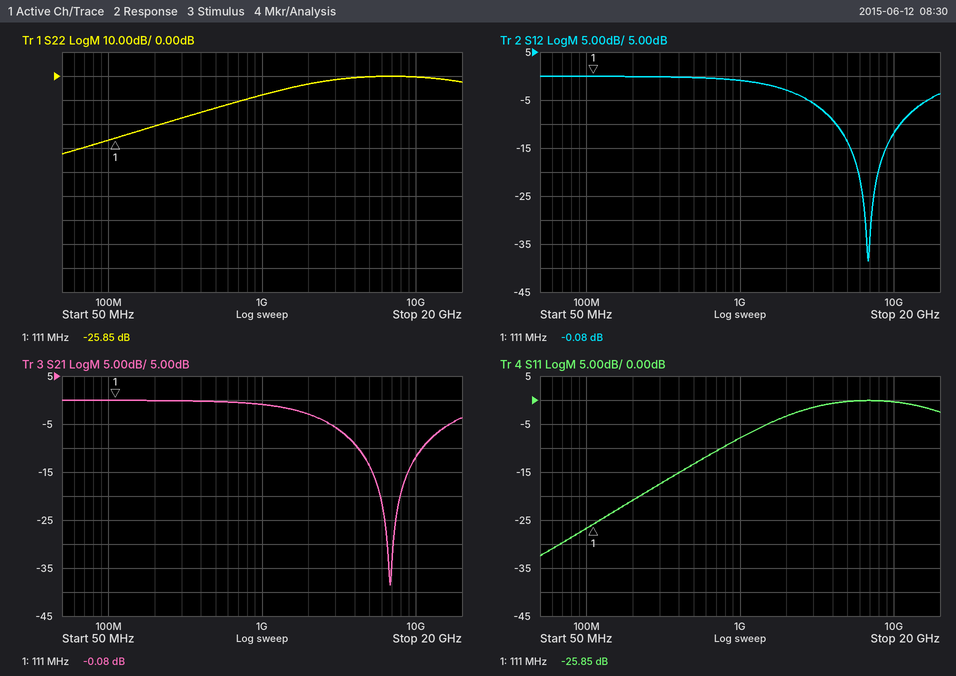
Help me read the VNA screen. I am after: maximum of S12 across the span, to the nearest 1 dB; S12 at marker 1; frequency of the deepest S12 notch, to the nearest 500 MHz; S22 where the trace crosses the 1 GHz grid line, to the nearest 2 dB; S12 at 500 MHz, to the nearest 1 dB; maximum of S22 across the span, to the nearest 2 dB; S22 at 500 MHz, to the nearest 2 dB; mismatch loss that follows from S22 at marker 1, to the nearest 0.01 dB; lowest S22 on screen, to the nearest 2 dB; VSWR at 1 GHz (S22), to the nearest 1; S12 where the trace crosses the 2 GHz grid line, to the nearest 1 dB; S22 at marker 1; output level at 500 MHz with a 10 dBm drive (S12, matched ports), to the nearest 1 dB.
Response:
0 dB
-0.08 dB
7.0 GHz
-8 dB
0 dB
0 dB
-14 dB
0.01 dB
-32 dB
2
-3 dB
-25.85 dB
10 dBm
